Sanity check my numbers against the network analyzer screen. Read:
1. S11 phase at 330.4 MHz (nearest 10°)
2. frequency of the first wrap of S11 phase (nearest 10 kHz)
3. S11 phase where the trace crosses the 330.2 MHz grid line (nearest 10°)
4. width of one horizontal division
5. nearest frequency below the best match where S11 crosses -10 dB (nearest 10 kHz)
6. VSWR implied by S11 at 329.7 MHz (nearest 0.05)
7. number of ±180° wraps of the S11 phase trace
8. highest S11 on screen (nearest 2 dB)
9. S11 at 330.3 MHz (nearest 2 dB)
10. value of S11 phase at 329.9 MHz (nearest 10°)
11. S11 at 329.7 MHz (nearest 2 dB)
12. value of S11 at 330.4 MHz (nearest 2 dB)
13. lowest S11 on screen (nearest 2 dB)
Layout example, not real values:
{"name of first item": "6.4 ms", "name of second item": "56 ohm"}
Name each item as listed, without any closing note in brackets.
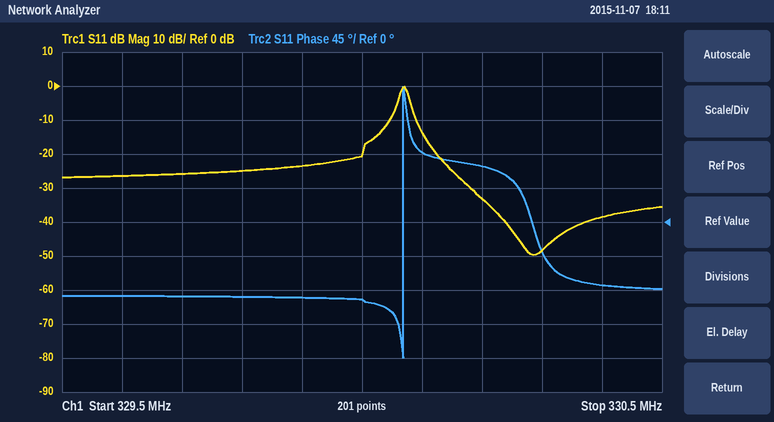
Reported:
{"S11 phase at 330.4 MHz": "-80°", "frequency of the first wrap of S11 phase": "330.07 MHz", "S11 phase where the trace crosses the 330.2 MHz grid line": "70°", "width of one horizontal division": "100 kHz", "nearest frequency below the best match where S11 crosses -10 dB": "330.09 MHz", "VSWR implied by S11 at 329.7 MHz": "1.10", "number of ±180° wraps of the S11 phase trace": "1", "highest S11 on screen": "0 dB", "S11 at 330.3 MHz": "-48 dB", "value of S11 phase at 329.9 MHz": "-100°", "S11 at 329.7 MHz": "-26 dB", "value of S11 at 330.4 MHz": "-38 dB", "lowest S11 on screen": "-50 dB"}
